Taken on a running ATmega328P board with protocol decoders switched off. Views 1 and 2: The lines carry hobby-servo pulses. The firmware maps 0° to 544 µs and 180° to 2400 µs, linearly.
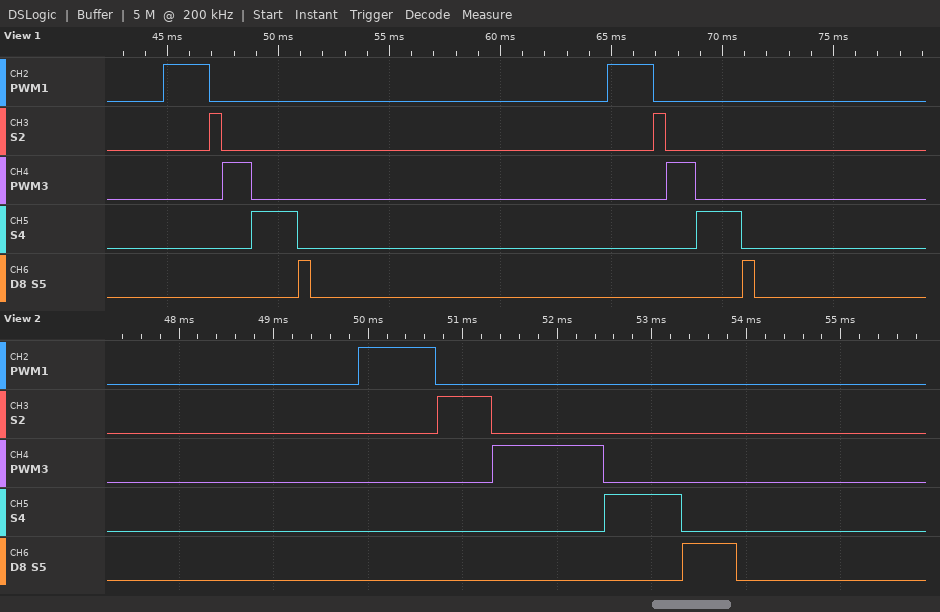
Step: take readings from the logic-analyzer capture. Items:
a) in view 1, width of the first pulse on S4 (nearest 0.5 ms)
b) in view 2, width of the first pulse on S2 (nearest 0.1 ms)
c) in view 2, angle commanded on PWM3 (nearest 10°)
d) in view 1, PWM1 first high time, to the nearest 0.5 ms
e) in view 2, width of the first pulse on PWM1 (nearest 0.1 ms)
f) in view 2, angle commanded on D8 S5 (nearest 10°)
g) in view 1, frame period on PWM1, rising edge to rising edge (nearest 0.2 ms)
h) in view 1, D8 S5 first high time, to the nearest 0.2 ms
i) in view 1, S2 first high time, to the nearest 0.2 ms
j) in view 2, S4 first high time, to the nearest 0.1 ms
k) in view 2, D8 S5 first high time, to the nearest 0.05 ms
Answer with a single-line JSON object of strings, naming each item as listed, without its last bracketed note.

{"in view 1, width of the first pulse on S4": "2.0 ms", "in view 2, width of the first pulse on S2": "0.6 ms", "in view 2, angle commanded on PWM3": "60°", "in view 1, PWM1 first high time, to the nearest 0.5 ms": "2.0 ms", "in view 2, width of the first pulse on PWM1": "0.8 ms", "in view 2, angle commanded on D8 S5": "0°", "in view 1, frame period on PWM1, rising edge to rising edge": "20.0 ms", "in view 1, D8 S5 first high time, to the nearest 0.2 ms": "0.6 ms", "in view 1, S2 first high time, to the nearest 0.2 ms": "0.6 ms", "in view 2, S4 first high time, to the nearest 0.1 ms": "0.8 ms", "in view 2, D8 S5 first high time, to the nearest 0.05 ms": "0.55 ms"}
